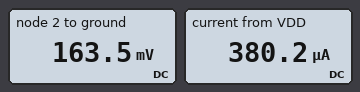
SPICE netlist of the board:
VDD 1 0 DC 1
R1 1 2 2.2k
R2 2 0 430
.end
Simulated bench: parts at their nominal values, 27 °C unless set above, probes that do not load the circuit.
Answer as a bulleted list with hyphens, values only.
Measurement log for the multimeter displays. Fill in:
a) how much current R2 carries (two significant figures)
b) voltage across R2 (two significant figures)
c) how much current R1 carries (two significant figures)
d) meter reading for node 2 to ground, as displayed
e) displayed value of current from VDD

- 380 µA
- 160 mV
- 380 µA
- 163.5 mV
- 380.2 µA
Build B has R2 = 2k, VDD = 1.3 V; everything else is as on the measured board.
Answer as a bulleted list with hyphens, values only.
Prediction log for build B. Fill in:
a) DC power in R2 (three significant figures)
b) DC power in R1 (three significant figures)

- 192 µW
- 211 µW
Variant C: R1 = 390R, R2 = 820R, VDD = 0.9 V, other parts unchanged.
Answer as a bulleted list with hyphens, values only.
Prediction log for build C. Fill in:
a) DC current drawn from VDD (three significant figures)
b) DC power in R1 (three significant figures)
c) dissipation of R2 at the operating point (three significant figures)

- 744 µA
- 216 µW
- 454 µW
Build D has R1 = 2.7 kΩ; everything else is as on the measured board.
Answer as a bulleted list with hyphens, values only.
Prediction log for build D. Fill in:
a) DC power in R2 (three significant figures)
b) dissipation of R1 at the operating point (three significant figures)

- 43.9 µW
- 276 µW
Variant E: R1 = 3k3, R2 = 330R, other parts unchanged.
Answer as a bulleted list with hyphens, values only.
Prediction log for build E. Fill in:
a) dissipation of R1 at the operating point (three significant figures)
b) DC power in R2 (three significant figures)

- 250 µW
- 25.0 µW
